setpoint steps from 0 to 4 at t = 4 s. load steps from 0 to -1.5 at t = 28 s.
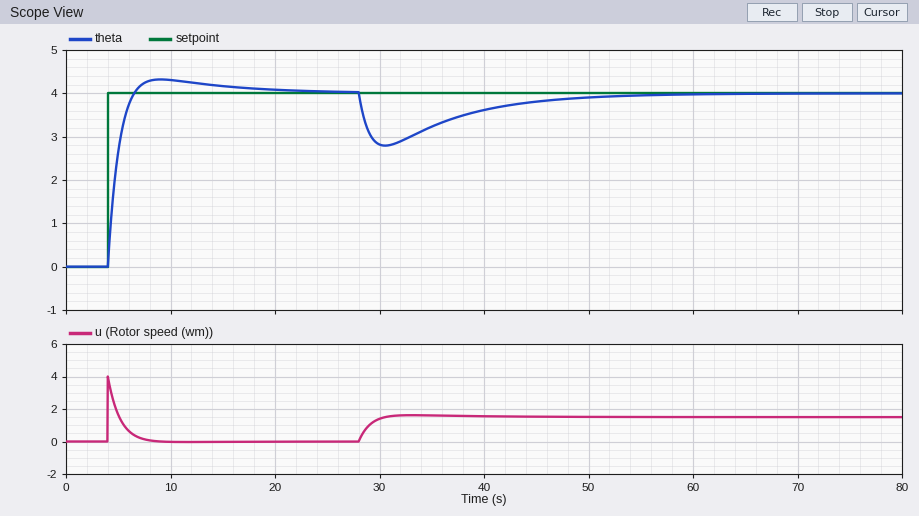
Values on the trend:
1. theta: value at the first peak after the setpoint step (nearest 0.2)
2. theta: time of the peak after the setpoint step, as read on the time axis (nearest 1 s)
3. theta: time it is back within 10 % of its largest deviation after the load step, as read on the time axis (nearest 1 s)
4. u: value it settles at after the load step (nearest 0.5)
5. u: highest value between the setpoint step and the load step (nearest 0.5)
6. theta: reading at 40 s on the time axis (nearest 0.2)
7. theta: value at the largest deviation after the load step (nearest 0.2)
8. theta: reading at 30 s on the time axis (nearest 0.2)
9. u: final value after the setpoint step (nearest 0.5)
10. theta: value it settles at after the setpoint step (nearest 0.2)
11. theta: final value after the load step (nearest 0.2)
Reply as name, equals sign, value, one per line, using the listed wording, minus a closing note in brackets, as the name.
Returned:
theta: value at the first peak after the setpoint step = 4.4
theta: time of the peak after the setpoint step, as read on the time axis = 9 s
theta: time it is back within 10 % of its largest deviation after the load step, as read on the time axis = 48 s
u: value it settles at after the load step = 1.5
u: highest value between the setpoint step and the load step = 4.0
theta: reading at 40 s on the time axis = 3.6
theta: value at the largest deviation after the load step = 2.8
theta: reading at 30 s on the time axis = 2.8
u: final value after the setpoint step = 0.0
theta: value it settles at after the setpoint step = 4.0
theta: final value after the load step = 4.0
